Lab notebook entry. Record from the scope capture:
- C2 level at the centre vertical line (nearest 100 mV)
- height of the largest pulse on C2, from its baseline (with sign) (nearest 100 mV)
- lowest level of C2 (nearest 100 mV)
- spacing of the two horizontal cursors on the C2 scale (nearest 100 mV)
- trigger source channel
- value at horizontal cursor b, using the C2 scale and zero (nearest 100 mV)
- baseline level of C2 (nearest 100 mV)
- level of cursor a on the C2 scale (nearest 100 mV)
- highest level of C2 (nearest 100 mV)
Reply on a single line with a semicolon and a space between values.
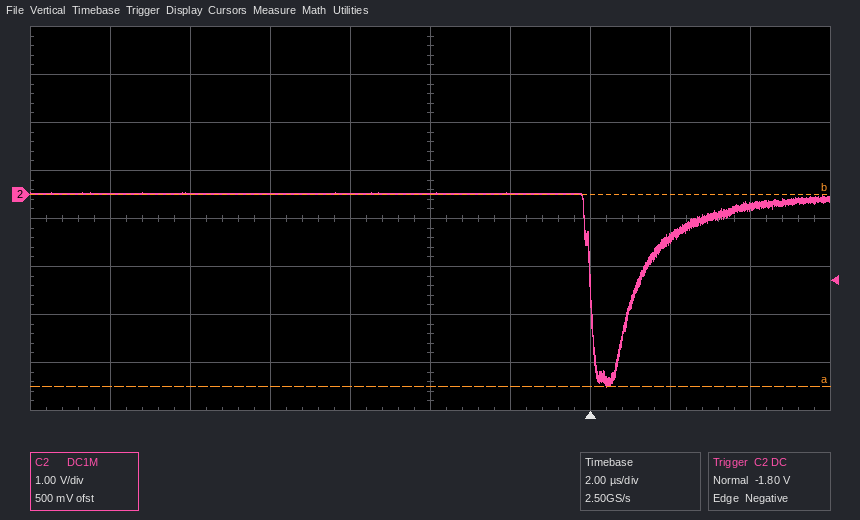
0.0 V; -4.0 V; -4.0 V; 4.0 V; C2; 0.0 V; 0.0 V; -4.0 V; 0.0 V
